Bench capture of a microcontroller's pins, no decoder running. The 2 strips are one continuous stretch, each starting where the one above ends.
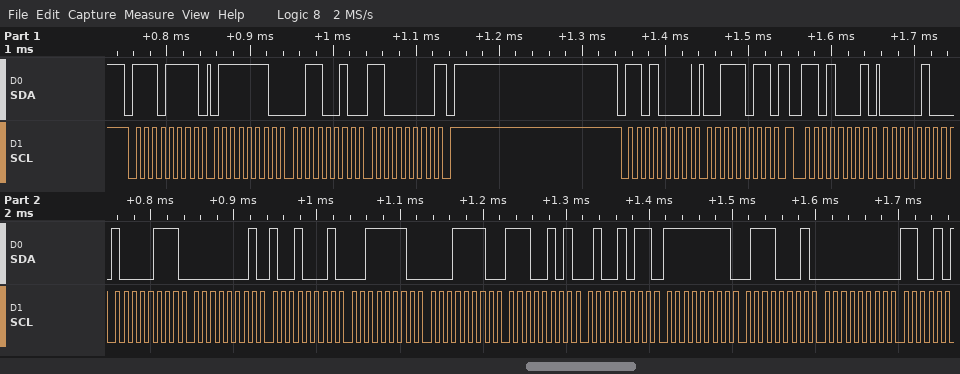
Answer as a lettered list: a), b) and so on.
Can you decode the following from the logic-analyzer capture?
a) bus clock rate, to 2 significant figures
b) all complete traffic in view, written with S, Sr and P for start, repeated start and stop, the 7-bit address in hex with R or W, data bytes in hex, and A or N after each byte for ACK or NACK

a) 100 kHz
b) S 77R A 7E A 32 A C0 N P S 68W A 3B A Sr 68R A 04 A 87 A 01 A 91 A 3E A 1E A E5 A 4B A FF A 71 A 00 A
